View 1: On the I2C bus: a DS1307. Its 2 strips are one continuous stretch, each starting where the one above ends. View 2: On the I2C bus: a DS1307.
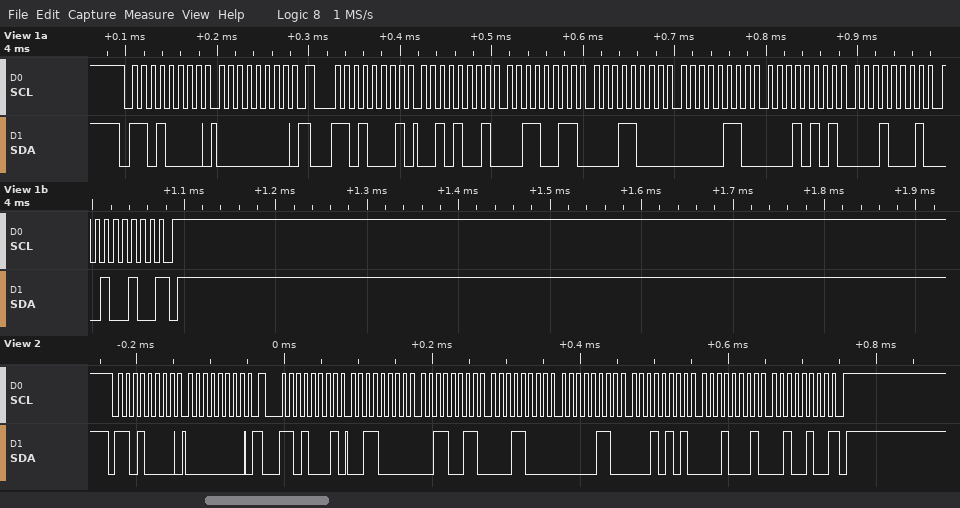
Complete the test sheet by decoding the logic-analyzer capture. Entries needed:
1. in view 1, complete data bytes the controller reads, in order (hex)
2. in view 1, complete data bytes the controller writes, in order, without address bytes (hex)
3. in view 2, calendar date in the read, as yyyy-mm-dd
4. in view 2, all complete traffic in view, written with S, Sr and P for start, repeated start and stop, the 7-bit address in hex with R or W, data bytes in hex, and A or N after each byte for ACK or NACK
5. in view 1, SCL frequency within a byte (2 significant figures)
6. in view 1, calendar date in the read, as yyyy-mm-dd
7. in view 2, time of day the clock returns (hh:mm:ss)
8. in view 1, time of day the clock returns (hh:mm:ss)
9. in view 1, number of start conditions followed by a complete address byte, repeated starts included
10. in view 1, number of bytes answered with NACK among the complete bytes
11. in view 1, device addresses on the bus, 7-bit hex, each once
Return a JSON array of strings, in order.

["29 33 18 06 15 11 24", "00", "2024-11-15", "S 68W A 00 A Sr 68R A 30 A 33 A 18 A 06 A 15 A 11 A 24 N P", "100 kHz", "2024-11-15", "18:33:30", "18:33:29", "2", "1", "0x68"]
